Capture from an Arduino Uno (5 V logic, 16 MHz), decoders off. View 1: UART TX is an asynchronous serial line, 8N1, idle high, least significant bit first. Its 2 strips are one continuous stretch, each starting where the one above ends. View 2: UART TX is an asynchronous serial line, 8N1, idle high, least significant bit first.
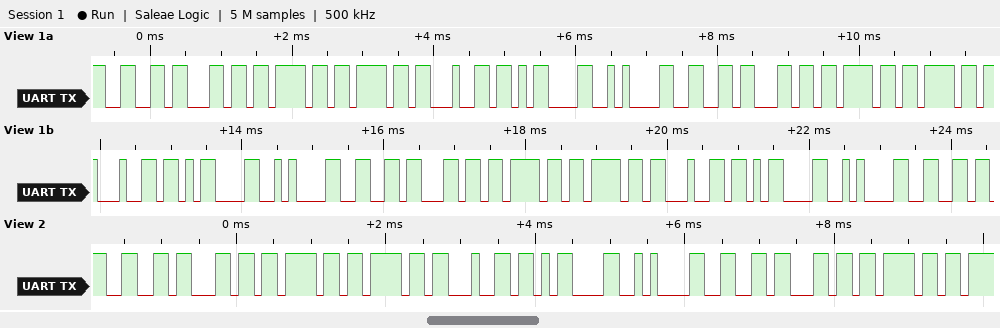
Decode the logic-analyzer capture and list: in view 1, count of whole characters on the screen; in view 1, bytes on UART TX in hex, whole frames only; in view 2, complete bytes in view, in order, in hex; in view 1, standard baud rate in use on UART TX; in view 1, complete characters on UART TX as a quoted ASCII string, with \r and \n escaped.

22
66 6C 6F 6F 64 0D 0A 66 6C 6F 6F 64 0D 0A 66 6C 6F 6F 64 0D 0A 66
66 6C 6F 6F 64 0D 0A 66 6C 6F
9600 baud
"flood\r\nflood\r\nflood\r\nf"
